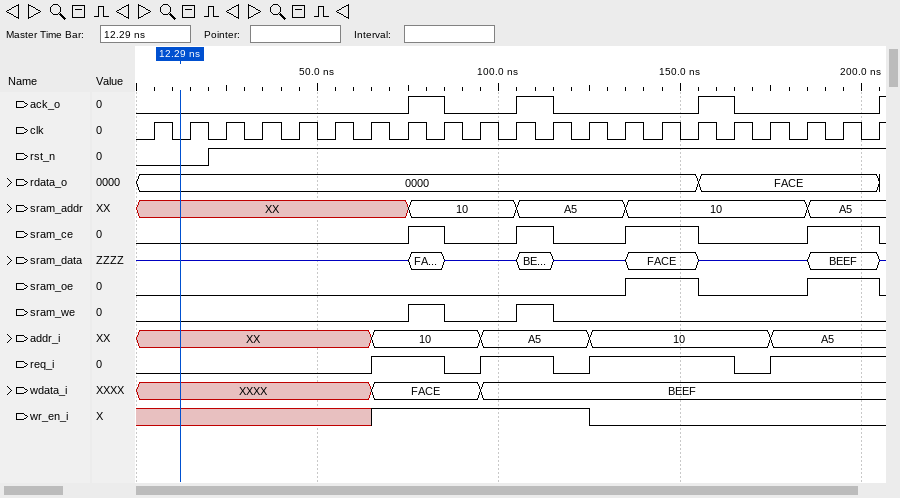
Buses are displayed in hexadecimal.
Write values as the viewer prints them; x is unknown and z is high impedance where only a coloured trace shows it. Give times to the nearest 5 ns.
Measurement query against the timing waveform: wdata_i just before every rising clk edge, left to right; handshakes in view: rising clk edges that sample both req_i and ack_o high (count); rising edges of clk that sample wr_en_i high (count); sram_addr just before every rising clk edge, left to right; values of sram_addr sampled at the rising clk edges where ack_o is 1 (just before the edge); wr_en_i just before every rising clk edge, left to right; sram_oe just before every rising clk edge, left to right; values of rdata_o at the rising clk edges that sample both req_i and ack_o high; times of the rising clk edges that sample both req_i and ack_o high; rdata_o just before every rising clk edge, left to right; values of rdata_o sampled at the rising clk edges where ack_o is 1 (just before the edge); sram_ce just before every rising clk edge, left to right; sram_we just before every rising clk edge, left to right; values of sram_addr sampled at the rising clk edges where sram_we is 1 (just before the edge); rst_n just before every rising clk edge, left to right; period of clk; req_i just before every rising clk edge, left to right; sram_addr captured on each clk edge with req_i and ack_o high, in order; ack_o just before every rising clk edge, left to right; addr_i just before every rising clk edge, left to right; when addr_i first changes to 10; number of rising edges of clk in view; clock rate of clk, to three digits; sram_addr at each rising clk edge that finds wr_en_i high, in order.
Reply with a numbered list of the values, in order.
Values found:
1. XXXX, XXXX, XXXX, XXXX, XXXX, XXXX, XXXX, FACE, FACE, FACE, BEEF, BEEF, BEEF, BEEF, BEEF, BEEF, BEEF, BEEF, BEEF, BEEF, BEEF
2. 3
3. 6
4. XX, XX, XX, XX, XX, XX, XX, XX, 10, 10, 10, A5, A5, A5, 10, 10, 10, 10, 10, A5, A5
5. 10, A5, 10
6. x x x x x x x 1 1 1 1 1 1 0 0 0 0 0 0 0 0
7. 0 0 0 0 0 0 0 0 0 0 0 0 0 0 1 1 0 0 0 1 1
8. 0000, 0000, FACE
9. 85 ns, 115 ns, 165 ns
10. 0000, 0000, 0000, 0000, 0000, 0000, 0000, 0000, 0000, 0000, 0000, 0000, 0000, 0000, 0000, 0000, FACE, FACE, FACE, FACE, FACE
11. 0000, 0000, FACE
12. 0 0 0 0 0 0 0 0 1 0 0 1 0 0 1 1 0 0 0 1 1
13. 0 0 0 0 0 0 0 0 1 0 0 1 0 0 0 0 0 0 0 0 0
14. 10, A5
15. 0 0 1 1 1 1 1 1 1 1 1 1 1 1 1 1 1 1 1 1 1
16. 10 ns
17. 0 0 0 0 0 0 0 1 1 0 1 1 0 1 1 1 1 0 1 1 1
18. 10, A5, 10
19. 0 0 0 0 0 0 0 0 1 0 0 1 0 0 0 0 1 0 0 0 0
20. XX, XX, XX, XX, XX, XX, XX, 10, 10, 10, A5, A5, A5, 10, 10, 10, 10, 10, A5, A5, A5
21. 65 ns
22. 21
23. 100 MHz
24. XX, 10, 10, 10, A5, A5
